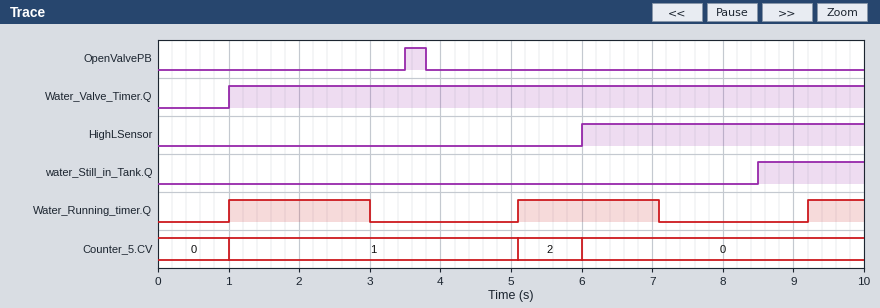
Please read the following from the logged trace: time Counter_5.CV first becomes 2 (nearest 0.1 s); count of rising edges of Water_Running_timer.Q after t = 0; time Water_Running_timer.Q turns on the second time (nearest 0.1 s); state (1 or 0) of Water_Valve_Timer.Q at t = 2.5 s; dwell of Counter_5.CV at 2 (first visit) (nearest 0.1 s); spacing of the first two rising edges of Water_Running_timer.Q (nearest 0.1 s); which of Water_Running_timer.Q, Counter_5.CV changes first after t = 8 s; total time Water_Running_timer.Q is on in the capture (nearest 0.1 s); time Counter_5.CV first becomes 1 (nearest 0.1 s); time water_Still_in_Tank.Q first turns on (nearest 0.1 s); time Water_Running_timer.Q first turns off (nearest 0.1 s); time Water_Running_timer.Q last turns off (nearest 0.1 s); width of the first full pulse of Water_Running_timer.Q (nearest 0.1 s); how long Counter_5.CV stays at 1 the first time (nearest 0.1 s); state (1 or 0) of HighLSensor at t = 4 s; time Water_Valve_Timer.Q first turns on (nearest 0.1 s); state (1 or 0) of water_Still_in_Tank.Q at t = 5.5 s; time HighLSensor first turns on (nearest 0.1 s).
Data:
5.1 s
3
5.1 s
1
0.9 s
4.1 s
Water_Running_timer.Q
4.8 s
1.0 s
8.5 s
3.0 s
7.1 s
2.0 s
4.1 s
0
1.0 s
0
6.0 s
